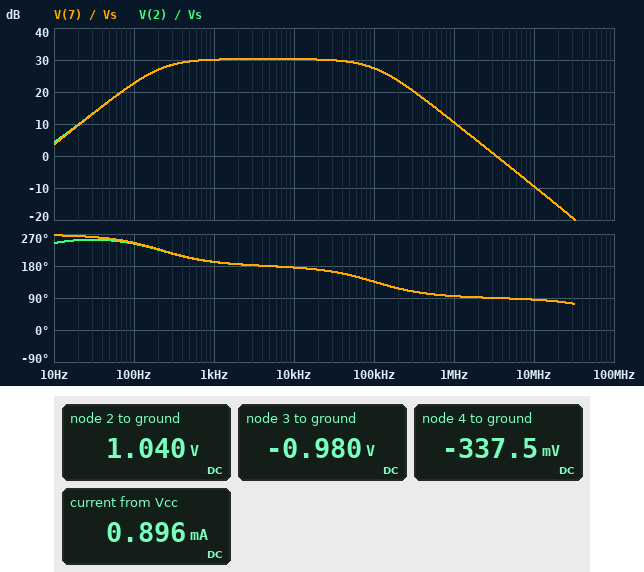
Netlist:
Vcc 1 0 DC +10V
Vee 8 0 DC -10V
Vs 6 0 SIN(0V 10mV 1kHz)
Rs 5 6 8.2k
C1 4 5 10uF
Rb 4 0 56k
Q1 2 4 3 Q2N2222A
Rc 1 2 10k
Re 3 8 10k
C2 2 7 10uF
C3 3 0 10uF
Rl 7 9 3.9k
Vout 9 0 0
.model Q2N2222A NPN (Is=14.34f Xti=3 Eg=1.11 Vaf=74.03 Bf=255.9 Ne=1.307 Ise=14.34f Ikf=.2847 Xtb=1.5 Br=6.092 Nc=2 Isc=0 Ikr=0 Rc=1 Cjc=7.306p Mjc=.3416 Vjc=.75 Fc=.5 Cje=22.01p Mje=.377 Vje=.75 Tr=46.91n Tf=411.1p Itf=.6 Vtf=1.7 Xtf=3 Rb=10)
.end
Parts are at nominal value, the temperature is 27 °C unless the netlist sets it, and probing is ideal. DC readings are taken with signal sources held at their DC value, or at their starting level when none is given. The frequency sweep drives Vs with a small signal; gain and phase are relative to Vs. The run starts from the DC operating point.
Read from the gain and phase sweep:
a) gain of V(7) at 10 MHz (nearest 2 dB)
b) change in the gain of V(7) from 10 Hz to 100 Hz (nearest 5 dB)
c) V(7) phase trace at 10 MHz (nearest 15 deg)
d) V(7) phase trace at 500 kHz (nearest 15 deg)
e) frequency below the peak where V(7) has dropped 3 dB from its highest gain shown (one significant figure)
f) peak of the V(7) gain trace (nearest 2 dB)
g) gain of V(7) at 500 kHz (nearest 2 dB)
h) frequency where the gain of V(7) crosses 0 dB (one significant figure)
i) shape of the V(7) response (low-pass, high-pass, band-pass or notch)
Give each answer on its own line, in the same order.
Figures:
-10 dB
20 dB
90 deg
105 deg
200 Hz
30 dB
16 dB
3 MHz
band-pass
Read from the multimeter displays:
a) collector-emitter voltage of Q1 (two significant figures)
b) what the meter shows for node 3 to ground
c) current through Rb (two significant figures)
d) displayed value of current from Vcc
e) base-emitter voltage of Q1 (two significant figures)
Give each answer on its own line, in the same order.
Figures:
2.0 V
-0.980 V
6.0 µA
0.896 mA
640 mV
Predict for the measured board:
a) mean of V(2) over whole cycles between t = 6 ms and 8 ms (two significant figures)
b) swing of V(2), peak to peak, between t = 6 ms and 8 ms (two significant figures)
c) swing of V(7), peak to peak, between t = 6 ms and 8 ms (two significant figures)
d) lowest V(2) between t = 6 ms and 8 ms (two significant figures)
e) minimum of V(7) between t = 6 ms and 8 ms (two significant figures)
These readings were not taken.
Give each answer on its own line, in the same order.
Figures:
1.0 V
640 mV
640 mV
720 mV
-320 mV
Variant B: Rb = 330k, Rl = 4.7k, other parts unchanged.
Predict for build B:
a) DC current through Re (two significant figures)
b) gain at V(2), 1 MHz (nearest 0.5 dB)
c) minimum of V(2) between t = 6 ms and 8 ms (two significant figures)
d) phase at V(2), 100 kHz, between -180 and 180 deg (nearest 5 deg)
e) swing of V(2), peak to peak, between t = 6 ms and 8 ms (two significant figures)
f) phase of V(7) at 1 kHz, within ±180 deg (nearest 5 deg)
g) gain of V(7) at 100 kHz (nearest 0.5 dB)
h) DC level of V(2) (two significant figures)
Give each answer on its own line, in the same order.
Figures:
770 µA
12.5 dB
2.0 V
140 deg
730 mV
-170 deg
29.0 dB
2.4 V
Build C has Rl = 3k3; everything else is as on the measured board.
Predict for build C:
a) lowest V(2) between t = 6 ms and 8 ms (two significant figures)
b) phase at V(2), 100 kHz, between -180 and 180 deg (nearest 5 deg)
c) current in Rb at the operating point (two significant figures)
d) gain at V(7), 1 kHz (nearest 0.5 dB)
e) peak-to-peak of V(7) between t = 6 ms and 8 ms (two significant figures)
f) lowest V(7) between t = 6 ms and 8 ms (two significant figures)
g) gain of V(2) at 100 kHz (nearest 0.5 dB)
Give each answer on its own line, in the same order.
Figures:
750 mV
140 deg
6.0 µA
29.0 dB
570 mV
-290 mV
27.0 dB
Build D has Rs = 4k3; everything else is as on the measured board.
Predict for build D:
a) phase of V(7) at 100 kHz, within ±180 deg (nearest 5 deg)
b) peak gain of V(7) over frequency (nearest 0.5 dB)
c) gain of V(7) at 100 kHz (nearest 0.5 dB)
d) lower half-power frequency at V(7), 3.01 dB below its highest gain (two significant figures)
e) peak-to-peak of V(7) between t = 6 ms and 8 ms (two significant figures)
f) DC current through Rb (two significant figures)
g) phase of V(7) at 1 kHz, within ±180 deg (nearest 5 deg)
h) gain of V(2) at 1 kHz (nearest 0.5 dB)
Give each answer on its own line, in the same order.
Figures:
145 deg
33.5 dB
31.5 dB
290 Hz
910 mV
6.0 µA
-165 deg
33.0 dB
